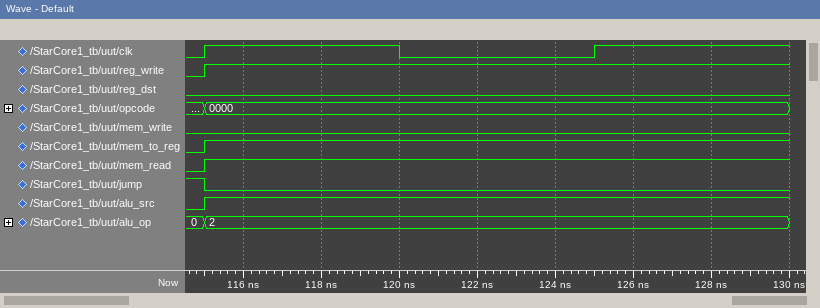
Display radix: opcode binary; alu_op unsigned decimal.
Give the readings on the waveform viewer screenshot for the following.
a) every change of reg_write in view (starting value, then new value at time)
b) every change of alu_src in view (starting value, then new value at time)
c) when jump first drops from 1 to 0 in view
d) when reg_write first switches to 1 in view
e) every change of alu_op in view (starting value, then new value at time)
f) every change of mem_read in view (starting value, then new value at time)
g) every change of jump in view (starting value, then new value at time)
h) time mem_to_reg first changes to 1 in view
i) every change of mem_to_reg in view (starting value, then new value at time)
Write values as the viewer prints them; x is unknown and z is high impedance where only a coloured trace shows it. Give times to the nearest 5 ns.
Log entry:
0, 1 at 115 ns
0, 1 at 115 ns
115 ns
115 ns
0, 2 at 115 ns
0, 1 at 115 ns
1, 0 at 115 ns
115 ns
0, 1 at 115 ns
